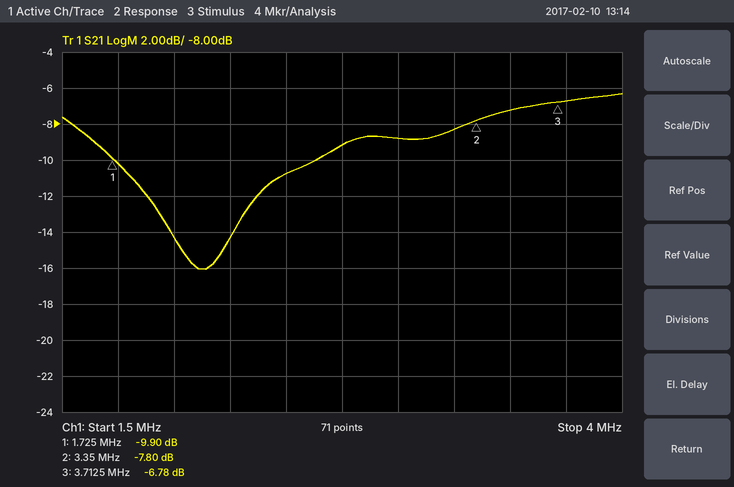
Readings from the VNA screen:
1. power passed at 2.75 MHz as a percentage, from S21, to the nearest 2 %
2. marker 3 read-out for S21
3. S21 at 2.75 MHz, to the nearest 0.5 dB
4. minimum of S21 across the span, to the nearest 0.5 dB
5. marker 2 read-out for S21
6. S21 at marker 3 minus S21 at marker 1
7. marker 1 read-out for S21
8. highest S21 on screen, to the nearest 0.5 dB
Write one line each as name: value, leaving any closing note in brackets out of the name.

power passed at 2.75 MHz as a percentage, from S21, to the nearest 2 %: 12 %
marker 3 read-out for S21: -6.78 dB
S21 at 2.75 MHz, to the nearest 0.5 dB: -9.0 dB
minimum of S21 across the span, to the nearest 0.5 dB: -16.0 dB
marker 2 read-out for S21: -7.80 dB
S21 at marker 3 minus S21 at marker 1: 3.12 dB
marker 1 read-out for S21: -9.90 dB
highest S21 on screen, to the nearest 0.5 dB: -6.5 dB
